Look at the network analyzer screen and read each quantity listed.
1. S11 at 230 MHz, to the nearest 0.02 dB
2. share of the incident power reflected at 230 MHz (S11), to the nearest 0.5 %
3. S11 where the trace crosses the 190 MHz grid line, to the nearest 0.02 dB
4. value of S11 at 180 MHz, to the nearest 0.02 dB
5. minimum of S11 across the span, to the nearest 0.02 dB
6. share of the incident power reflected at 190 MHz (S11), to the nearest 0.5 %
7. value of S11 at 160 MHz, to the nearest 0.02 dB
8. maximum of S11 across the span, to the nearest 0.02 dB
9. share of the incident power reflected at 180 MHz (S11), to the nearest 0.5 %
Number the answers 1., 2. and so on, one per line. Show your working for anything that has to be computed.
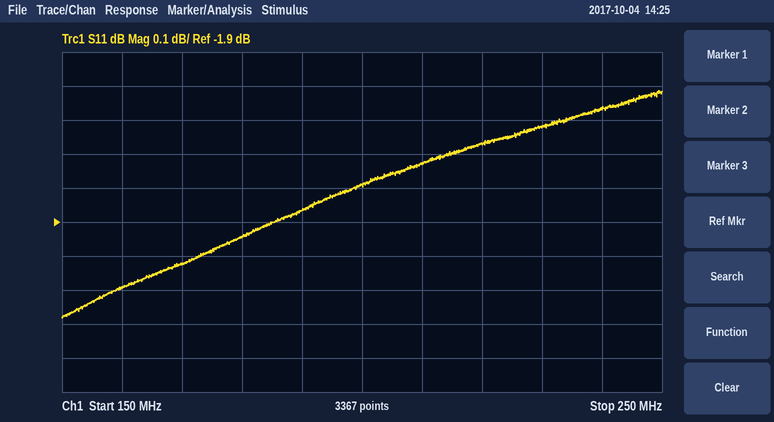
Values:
1. -1.62 dB
2. 10^(-1.62/10) ≈ 68.9 %, so 69.0 % to the nearest 0.5 %
3. -1.86 dB
4. -1.94 dB
5. -2.18 dB
6. 10^(-1.86/10) ≈ 65.2 %, so 65.0 % to the nearest 0.5 %
7. -2.10 dB
8. -1.52 dB
9. 10^(-1.94/10) ≈ 64.0 %
